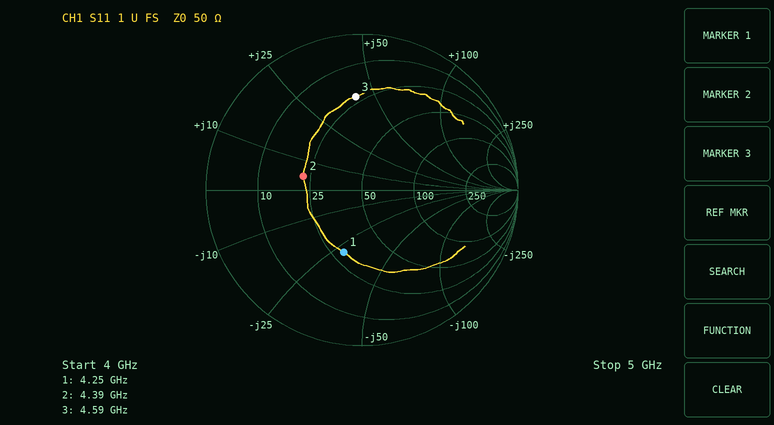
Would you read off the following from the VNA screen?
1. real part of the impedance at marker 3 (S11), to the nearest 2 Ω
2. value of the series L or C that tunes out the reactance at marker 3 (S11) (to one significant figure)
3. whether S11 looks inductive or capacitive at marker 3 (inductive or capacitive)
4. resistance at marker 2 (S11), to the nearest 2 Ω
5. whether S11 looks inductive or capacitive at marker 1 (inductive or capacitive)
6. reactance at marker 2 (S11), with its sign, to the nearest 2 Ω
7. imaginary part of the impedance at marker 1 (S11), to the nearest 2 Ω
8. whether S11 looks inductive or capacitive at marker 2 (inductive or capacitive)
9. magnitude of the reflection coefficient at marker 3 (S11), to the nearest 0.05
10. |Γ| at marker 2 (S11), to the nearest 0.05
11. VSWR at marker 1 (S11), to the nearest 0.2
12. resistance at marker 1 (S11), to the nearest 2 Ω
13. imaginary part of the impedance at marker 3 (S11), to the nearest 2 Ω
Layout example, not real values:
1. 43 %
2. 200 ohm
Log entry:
1. 22 Ω
2. 800 fF
3. inductive
4. 22 Ω
5. capacitive
6. +4 Ω
7. -28 Ω
8. inductive
9. 0.60
10. 0.40
11. 2.4
12. 30 Ω
13. +42 Ω
